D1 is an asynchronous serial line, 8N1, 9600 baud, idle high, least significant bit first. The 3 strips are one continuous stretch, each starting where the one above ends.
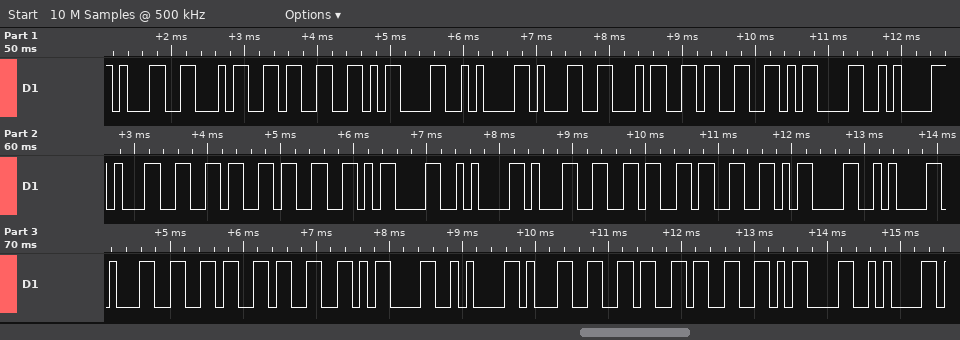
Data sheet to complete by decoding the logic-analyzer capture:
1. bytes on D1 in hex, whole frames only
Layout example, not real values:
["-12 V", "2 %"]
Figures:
["31 34 33 0D 0A 31 34 33 0D 0A 31 36 33 0D 0A 31 36 33 0D 0A 31 36 33 0D 0A 31 36 33 0D 0A"]
